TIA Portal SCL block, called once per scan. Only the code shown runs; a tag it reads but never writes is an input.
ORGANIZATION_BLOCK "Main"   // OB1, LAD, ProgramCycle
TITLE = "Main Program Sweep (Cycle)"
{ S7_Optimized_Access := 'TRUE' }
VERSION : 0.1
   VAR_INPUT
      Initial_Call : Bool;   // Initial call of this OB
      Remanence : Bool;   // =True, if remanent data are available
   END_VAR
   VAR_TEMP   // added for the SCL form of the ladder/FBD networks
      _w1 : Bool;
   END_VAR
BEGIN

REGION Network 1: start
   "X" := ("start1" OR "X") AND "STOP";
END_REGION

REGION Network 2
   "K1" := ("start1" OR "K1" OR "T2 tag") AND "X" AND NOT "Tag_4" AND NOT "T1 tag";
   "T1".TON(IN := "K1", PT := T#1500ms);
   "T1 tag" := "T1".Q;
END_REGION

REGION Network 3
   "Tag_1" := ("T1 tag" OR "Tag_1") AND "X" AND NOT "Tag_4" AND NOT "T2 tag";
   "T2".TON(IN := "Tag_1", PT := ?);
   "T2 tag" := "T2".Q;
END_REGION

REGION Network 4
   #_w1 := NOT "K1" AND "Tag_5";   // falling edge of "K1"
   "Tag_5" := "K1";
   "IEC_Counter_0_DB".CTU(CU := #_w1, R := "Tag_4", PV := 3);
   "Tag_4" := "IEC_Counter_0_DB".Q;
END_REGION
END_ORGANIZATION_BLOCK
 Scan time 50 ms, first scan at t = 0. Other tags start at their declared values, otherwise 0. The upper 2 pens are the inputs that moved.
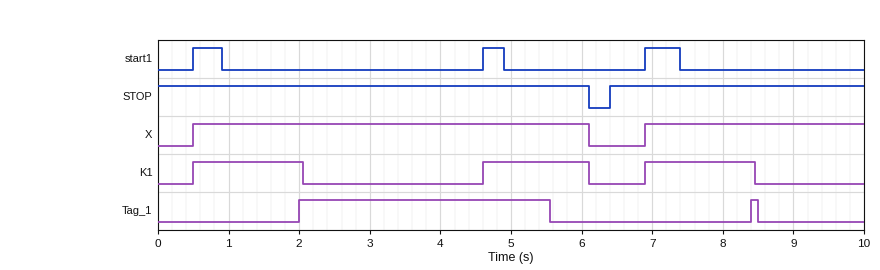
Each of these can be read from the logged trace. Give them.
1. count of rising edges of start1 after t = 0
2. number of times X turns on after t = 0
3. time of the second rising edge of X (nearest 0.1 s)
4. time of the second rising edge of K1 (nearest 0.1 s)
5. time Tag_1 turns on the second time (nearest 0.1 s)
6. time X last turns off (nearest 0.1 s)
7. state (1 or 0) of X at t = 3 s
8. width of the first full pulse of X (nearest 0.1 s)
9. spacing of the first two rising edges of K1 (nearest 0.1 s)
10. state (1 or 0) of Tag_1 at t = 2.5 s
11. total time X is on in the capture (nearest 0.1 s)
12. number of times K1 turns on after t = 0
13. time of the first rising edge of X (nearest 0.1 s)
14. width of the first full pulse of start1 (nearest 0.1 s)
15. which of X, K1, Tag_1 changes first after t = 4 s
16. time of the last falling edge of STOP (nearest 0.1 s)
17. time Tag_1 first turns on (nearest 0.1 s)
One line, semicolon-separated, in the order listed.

3; 2; 6.9 s; 4.6 s; 8.4 s; 6.1 s; 1; 5.6 s; 4.1 s; 1; 8.7 s; 3; 0.5 s; 0.4 s; K1; 6.1 s; 2.0 s
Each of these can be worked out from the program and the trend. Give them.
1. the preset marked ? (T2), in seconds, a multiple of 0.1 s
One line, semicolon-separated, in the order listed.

3.5 s
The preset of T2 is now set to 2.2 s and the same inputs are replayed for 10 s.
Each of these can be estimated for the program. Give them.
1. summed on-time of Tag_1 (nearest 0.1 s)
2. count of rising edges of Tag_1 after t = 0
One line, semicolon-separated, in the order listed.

2.7 s; 3
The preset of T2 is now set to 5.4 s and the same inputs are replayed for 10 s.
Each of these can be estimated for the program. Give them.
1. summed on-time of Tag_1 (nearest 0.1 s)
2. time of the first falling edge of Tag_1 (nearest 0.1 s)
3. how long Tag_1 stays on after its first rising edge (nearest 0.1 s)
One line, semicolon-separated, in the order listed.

4.2 s; 6.1 s; 4.1 s
